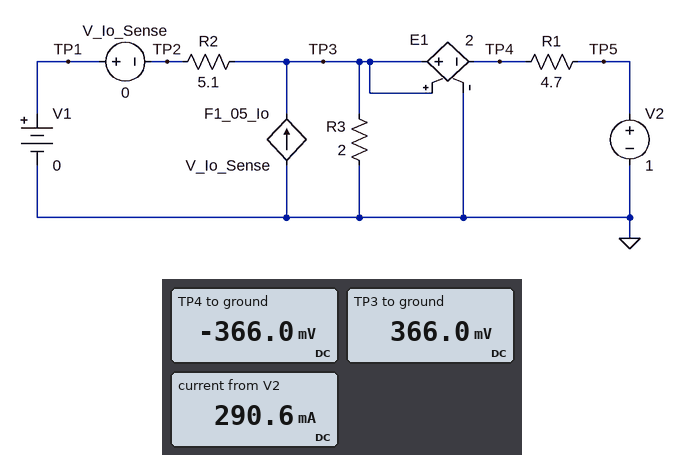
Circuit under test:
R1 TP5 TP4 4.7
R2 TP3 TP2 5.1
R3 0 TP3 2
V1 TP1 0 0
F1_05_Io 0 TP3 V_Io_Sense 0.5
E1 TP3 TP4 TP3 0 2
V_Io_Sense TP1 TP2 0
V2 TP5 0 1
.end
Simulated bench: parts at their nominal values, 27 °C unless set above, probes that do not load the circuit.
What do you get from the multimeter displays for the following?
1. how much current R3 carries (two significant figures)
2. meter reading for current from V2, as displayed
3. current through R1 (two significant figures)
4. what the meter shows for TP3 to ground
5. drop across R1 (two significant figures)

180 mA
290.6 mA
290 mA
366.0 mV
1.4 V
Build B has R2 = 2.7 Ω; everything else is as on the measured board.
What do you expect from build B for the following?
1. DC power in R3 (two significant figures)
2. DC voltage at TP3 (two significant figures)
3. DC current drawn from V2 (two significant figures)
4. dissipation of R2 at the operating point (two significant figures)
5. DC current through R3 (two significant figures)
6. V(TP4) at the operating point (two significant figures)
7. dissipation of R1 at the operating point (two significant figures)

32 mW
250 mV
270 mA
24 mW
130 mA
-250 mV
330 mW
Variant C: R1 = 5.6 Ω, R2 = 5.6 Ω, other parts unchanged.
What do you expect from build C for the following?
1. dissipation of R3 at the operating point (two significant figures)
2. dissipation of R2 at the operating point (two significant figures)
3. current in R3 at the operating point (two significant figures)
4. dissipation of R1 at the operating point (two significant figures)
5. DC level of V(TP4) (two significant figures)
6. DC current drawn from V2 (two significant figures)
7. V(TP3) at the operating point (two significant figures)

46 mW
16 mW
150 mA
300 mW
-300 mV
230 mA
300 mV
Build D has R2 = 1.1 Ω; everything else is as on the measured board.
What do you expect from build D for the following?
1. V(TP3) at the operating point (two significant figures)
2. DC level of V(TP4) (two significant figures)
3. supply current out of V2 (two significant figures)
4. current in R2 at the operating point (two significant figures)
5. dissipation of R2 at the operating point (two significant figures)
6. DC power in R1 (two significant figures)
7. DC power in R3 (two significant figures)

130 mV
-130 mV
240 mA
120 mA
15 mW
270 mW
8.3 mW
